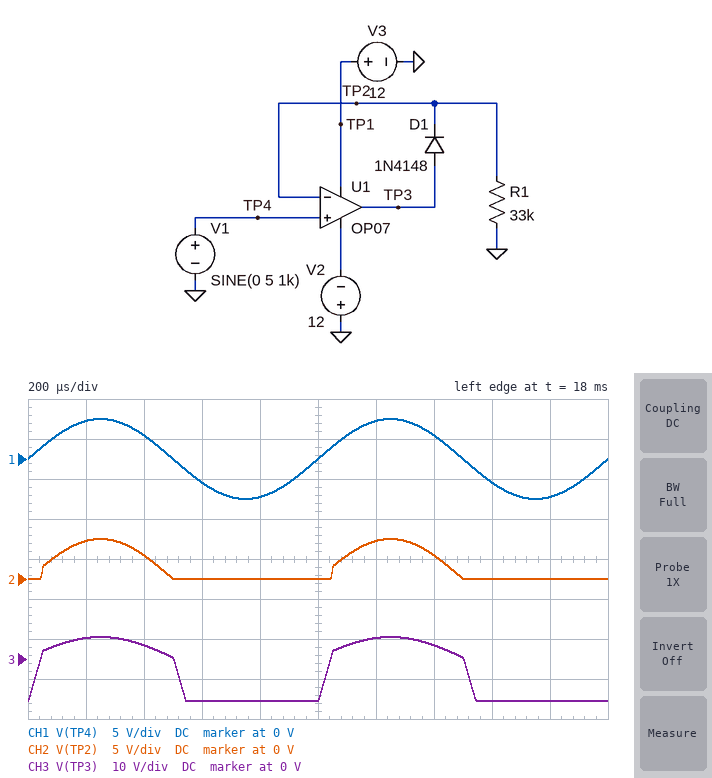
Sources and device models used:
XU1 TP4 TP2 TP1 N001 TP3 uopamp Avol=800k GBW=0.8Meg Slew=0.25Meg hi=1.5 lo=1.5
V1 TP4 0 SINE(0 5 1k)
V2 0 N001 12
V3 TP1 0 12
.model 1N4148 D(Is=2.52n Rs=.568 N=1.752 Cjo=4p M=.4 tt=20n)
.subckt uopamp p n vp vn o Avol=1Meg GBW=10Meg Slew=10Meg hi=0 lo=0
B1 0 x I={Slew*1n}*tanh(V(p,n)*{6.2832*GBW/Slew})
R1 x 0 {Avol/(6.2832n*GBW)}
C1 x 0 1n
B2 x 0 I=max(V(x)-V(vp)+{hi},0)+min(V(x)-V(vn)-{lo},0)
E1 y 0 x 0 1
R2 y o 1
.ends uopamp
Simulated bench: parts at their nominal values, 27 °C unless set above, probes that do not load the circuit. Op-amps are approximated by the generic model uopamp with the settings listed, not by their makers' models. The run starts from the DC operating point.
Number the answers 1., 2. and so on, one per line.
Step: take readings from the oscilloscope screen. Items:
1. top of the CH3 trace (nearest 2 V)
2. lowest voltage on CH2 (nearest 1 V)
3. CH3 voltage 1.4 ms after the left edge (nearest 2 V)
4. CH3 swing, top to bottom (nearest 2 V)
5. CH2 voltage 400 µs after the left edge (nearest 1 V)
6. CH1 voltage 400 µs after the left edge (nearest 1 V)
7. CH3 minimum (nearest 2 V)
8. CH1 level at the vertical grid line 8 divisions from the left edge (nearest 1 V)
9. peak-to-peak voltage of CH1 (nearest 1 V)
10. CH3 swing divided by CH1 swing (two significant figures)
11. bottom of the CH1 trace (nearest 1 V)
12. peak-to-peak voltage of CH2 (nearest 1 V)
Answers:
1. 6 V
2. 0 V
3. 4 V
4. 16 V
5. 3 V
6. 3 V
7. -10 V
8. -3 V
9. 10 V
10. 1.6
11. -5 V
12. 5 V
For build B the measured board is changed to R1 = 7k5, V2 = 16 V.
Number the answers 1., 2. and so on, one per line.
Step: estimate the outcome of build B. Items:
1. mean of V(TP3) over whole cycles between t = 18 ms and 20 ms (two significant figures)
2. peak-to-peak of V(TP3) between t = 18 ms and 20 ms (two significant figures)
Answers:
1. -5.5 V
2. 20 V
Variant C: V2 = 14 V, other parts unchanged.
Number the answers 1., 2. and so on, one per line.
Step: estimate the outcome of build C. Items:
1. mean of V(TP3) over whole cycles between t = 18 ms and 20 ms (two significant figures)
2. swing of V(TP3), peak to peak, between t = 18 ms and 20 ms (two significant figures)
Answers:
1. -4.5 V
2. 18 V
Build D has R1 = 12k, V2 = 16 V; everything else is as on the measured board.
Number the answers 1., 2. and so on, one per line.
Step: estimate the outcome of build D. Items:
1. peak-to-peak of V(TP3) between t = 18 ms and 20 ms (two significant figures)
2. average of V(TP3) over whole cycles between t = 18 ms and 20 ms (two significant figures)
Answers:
1. 20 V
2. -5.5 V
